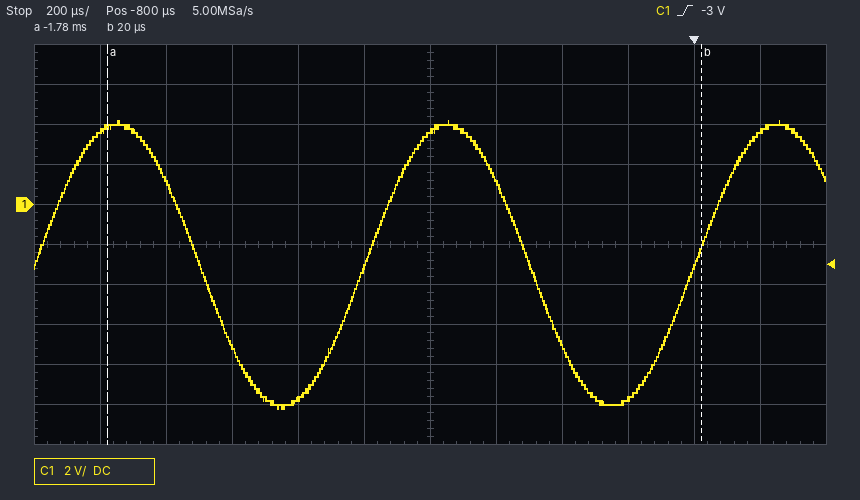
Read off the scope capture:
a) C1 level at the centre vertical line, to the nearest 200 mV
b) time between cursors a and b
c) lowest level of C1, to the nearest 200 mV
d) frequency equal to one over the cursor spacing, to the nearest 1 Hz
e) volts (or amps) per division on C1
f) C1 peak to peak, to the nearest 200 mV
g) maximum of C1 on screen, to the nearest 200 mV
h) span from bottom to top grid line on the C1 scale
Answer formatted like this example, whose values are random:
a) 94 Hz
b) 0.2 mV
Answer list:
a) 3.6 V
b) 1.80 ms
c) -10.2 V
d) 556 Hz
e) 2 V
f) 14.4 V
g) 4.2 V
h) 20 V
